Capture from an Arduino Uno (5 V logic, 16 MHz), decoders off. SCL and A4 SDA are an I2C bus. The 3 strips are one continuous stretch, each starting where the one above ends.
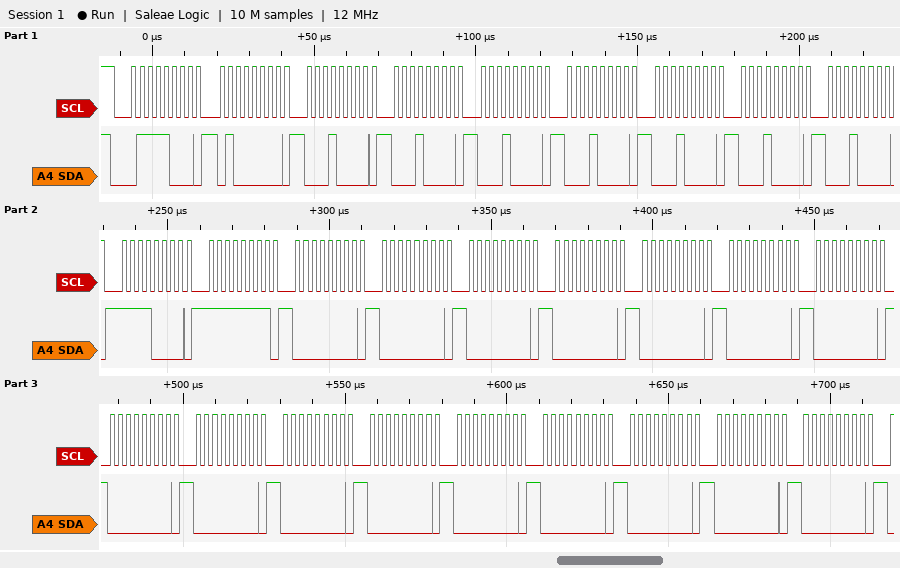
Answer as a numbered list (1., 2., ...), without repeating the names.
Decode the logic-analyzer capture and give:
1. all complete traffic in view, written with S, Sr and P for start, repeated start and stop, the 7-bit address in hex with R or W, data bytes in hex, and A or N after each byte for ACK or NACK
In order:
1. S 3CW A 40 A 10 A 10 A 10 A 10 A 10 A 10 A 10 A F0 A FF A 00 A 00 A 00 A 00 A 00 A 00 A 00 A 00 A 00 A 00 A 00 A 00 A 00 A 00 A 00 A 00 A
